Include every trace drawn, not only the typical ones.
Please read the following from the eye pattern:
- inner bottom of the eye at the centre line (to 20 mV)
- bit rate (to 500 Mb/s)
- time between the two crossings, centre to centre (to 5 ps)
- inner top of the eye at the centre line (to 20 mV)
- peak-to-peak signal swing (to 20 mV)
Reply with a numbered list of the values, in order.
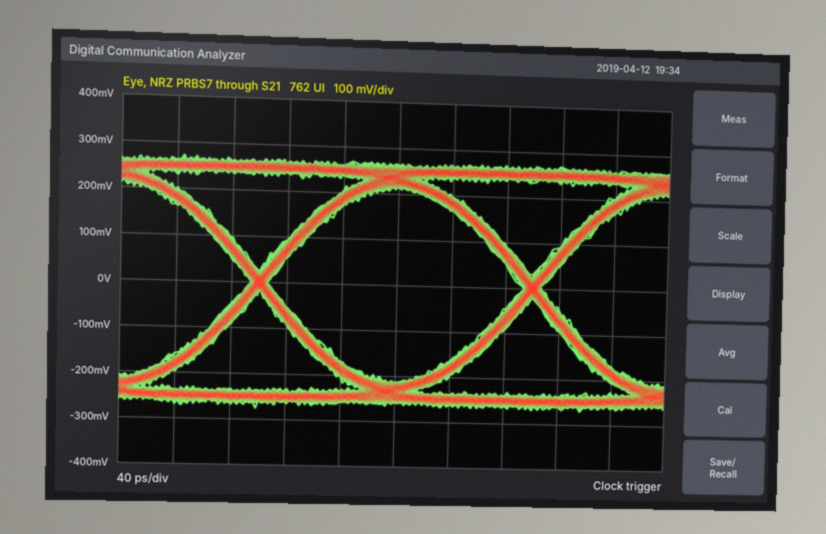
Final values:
1. -220 mV
2. 5.0 Gb/s
3. 200 ps
4. 220 mV
5. 540 mV
